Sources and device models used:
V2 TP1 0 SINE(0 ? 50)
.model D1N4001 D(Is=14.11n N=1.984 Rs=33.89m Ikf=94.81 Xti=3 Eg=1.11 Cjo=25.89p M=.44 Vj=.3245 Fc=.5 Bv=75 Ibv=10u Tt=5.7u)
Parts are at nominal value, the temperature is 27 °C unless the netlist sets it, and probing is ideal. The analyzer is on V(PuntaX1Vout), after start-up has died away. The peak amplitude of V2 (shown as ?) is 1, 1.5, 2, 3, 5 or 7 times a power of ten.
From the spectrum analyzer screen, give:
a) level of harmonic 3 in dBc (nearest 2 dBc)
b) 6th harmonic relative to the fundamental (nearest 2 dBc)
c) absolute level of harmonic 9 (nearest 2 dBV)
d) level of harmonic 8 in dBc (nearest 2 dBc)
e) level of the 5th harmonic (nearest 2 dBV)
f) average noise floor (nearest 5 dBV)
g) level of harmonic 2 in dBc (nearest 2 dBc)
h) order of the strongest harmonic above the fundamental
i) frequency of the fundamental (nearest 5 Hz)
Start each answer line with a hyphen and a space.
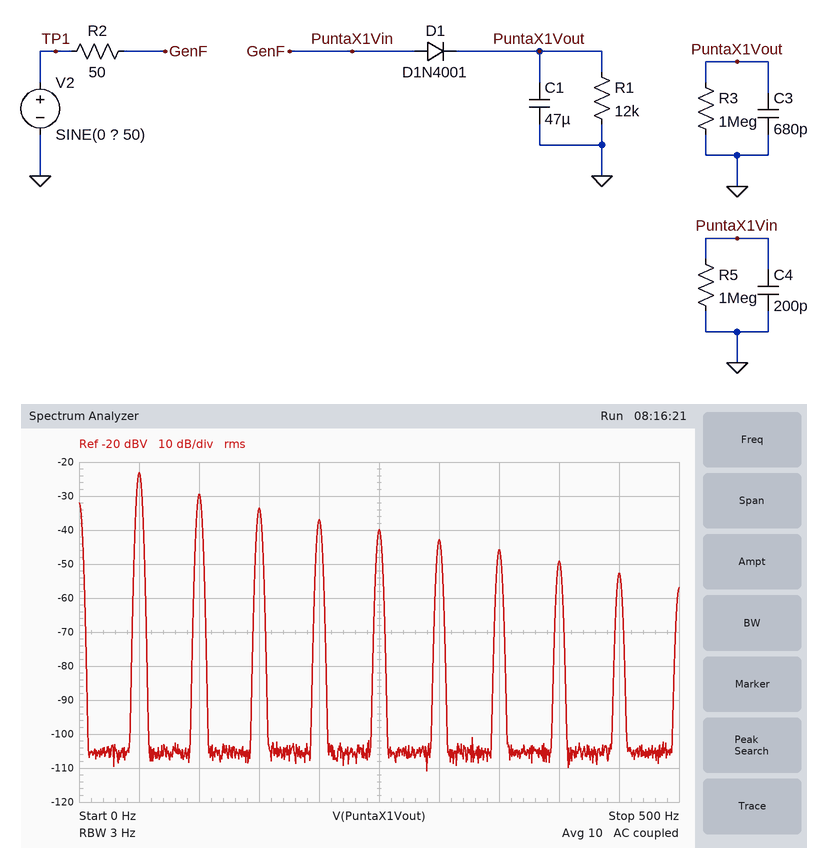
- -10 dBc
- -20 dBc
- -52 dBV
- -26 dBc
- -40 dBV
- -105 dBV
- -6 dBc
- 2
- 50 Hz
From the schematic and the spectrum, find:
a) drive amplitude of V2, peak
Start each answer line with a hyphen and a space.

- 10 V
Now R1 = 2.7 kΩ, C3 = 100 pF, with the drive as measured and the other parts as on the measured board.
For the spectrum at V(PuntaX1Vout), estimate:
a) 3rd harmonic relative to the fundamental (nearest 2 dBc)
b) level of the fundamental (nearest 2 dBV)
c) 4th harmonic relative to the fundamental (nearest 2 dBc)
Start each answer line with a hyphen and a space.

- -12 dBc
- -12 dBV
- -16 dBc
